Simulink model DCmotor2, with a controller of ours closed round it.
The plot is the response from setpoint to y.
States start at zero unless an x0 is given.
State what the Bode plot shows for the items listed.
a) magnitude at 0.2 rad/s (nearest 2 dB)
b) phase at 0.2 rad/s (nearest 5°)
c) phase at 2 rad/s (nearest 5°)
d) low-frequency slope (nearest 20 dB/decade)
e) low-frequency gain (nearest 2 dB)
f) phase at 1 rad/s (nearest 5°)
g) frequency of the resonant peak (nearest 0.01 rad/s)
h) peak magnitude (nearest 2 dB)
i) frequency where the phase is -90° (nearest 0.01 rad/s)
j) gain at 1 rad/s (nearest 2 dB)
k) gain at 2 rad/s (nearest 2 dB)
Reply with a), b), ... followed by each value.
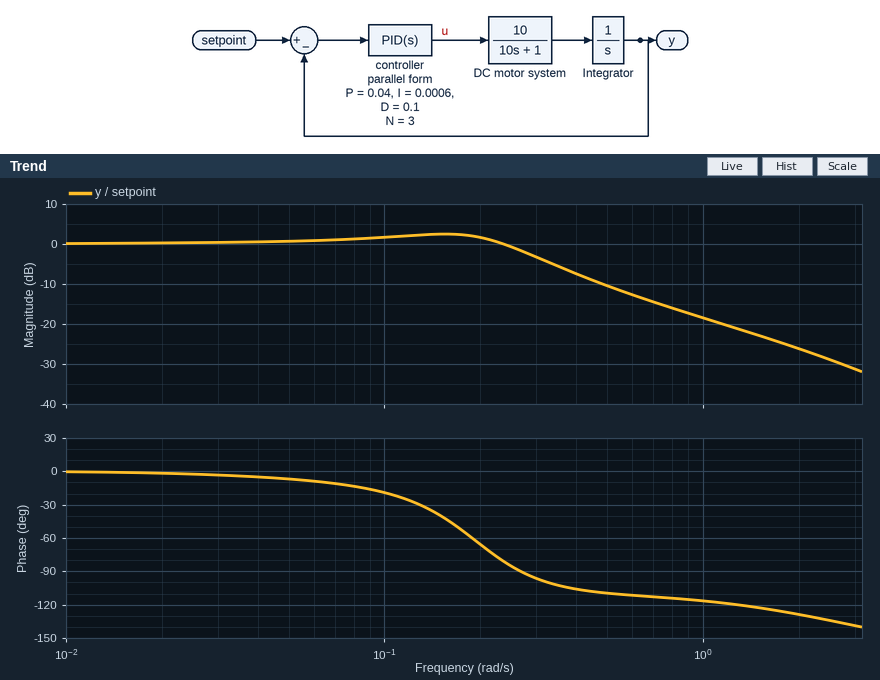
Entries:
a) 2 dB
b) -65°
c) -130°
d) 0 dB/decade
e) 0 dB
f) -115°
g) 0.15 rad/s
h) 2 dB
i) 0.27 rad/s
j) -18 dB
k) -26 dB
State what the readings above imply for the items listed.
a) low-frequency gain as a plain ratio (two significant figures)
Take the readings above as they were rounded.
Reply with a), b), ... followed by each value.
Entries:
a) 1.0
